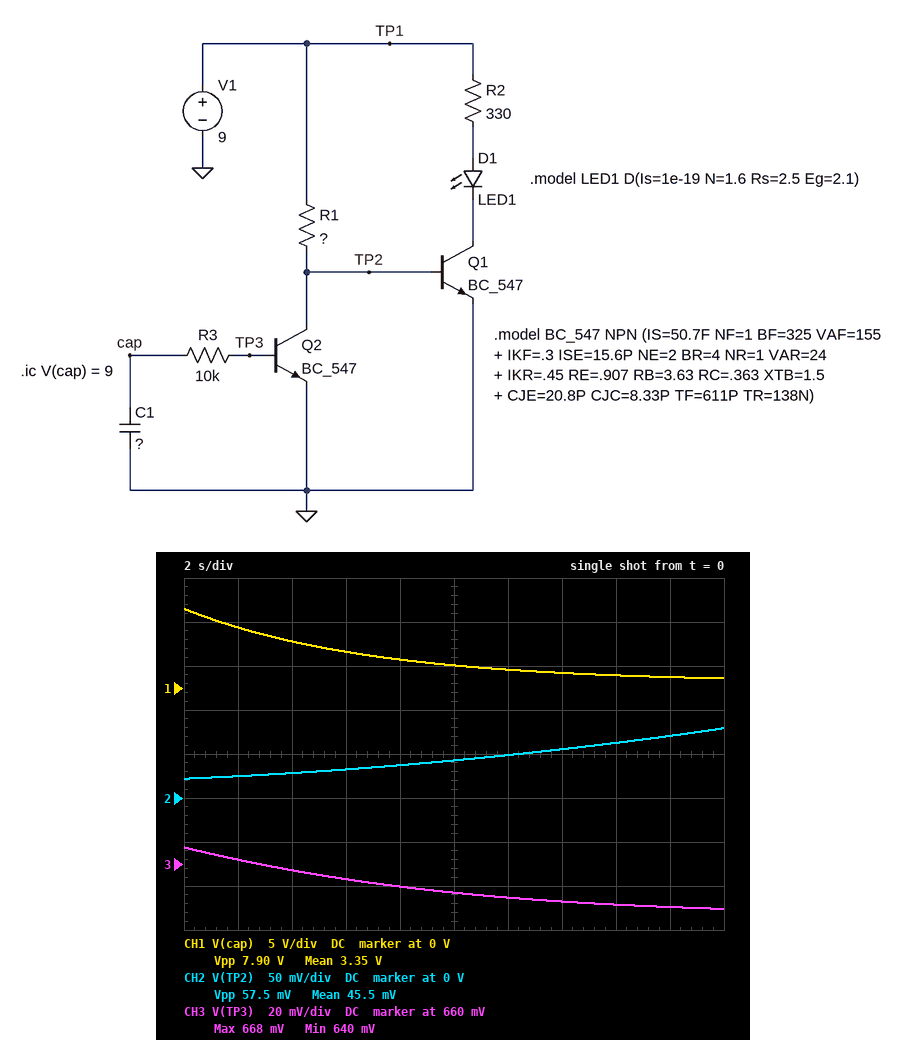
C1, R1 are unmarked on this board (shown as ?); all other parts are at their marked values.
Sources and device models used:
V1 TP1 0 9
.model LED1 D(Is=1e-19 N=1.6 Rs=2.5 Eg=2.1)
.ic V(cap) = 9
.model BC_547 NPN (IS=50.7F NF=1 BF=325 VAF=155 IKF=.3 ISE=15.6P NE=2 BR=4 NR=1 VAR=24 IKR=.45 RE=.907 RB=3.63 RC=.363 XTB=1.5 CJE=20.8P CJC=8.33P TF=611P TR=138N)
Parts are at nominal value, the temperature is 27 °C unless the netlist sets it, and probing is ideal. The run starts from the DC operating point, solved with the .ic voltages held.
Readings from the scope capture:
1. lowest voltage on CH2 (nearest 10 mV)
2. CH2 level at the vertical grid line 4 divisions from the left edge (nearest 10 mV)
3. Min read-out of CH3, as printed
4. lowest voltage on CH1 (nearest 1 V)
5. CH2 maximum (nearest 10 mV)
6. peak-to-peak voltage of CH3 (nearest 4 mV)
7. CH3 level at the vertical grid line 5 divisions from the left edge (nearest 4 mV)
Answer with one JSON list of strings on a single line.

["20 mV", "40 mV", "640 mV", "1 V", "80 mV", "28 mV", "648 mV"]
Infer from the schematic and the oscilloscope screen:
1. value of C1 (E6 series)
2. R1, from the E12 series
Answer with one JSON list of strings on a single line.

["680 µF", "3.9 kΩ"]
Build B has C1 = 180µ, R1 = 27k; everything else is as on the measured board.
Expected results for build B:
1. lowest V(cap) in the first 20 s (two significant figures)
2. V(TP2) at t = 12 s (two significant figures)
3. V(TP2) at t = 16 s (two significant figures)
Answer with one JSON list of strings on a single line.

["550 mV", "710 mV", "720 mV"]
